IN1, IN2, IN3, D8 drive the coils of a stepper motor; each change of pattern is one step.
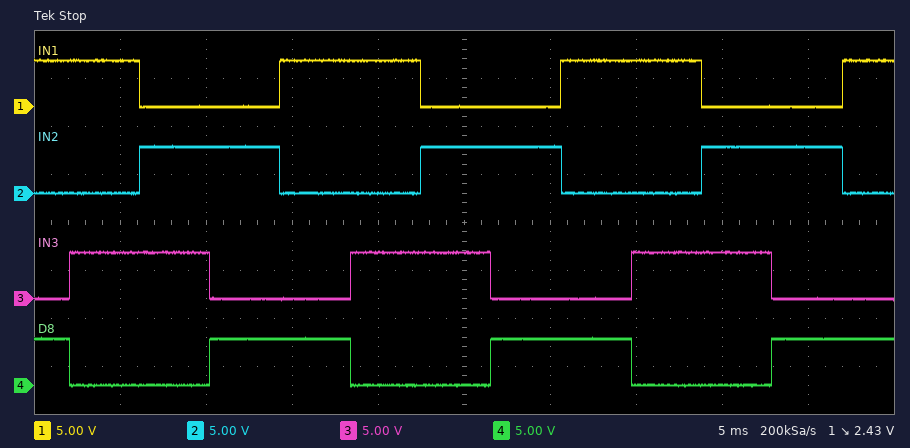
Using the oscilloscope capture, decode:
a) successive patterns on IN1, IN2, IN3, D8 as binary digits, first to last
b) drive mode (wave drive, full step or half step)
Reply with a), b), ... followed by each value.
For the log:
a) 1001 1010 0110 0101 1001 1010 0110 0101 1001 1010 0110 0101 1001
b) full step
